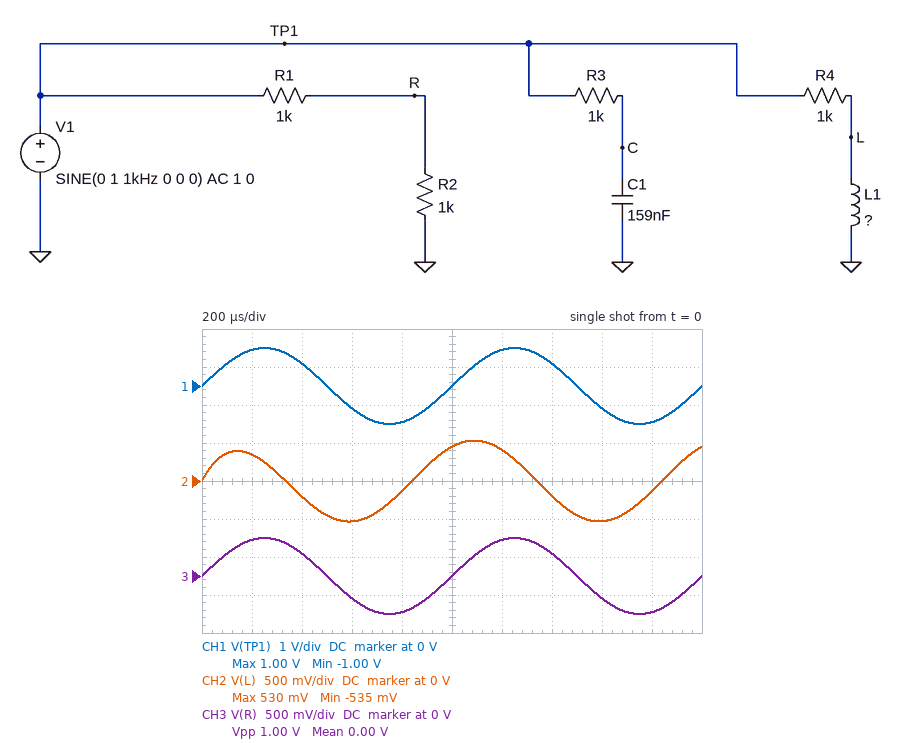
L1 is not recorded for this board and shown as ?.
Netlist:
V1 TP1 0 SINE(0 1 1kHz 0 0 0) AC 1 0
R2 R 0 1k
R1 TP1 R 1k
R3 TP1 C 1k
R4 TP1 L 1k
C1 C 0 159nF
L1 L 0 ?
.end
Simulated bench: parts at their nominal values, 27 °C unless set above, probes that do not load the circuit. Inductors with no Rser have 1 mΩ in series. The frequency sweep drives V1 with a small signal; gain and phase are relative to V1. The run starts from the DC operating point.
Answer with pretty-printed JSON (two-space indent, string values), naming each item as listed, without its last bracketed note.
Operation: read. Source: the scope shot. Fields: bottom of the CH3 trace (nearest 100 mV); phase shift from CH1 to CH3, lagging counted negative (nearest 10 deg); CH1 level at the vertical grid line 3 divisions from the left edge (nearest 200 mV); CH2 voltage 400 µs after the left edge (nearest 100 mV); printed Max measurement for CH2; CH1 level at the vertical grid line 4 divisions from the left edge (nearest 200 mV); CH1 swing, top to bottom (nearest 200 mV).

{
  "bottom of the CH3 trace": "-500 mV",
  "phase shift from CH1 to CH3, lagging counted negative": "0 deg",
  "CH1 level at the vertical grid line 3 divisions from the left edge": "-600 mV",
  "CH2 voltage 400 µs after the left edge": "-200 mV",
  "printed Max measurement for CH2": "530 mV",
  "CH1 level at the vertical grid line 4 divisions from the left edge": "-1.0 V",
  "CH1 swing, top to bottom": "2.0 V"
}
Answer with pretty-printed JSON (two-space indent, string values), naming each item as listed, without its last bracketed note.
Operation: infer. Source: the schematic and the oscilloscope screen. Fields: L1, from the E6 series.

{
  "L1, from the E6 series": "100 mH"
}
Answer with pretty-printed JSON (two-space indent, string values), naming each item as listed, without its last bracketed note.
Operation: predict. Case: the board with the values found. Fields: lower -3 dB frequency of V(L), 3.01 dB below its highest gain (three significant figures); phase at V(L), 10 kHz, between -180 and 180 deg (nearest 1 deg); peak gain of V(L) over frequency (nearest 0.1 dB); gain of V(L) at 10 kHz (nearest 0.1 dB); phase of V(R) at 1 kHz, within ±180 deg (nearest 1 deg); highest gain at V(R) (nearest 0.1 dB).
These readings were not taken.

{
  "lower -3 dB frequency of V(L), 3.01 dB below its highest gain": "1.59 kHz",
  "phase at V(L), 10 kHz, between -180 and 180 deg": "9 deg",
  "peak gain of V(L) over frequency": "0 dB",
  "gain of V(L) at 10 kHz": "-0.1 dB",
  "phase of V(R) at 1 kHz, within ±180 deg": "0 deg",
  "highest gain at V(R)": "-6.0 dB"
}
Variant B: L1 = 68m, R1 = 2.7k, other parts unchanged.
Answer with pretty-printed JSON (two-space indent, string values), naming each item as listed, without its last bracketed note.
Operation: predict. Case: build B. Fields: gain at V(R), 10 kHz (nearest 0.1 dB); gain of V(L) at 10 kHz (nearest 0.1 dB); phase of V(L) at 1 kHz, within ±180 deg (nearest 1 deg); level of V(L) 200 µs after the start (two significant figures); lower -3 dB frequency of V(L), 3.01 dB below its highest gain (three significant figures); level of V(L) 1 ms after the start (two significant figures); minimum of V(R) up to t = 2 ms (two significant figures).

{
  "gain at V(R), 10 kHz": "-11.4 dB",
  "gain of V(L) at 10 kHz": "-0.2 dB",
  "phase of V(L) at 1 kHz, within ±180 deg": "67 deg",
  "level of V(L) 200 µs after the start": "240 mV",
  "lower -3 dB frequency of V(L), 3.01 dB below its highest gain": "2.34 kHz",
  "level of V(L) 1 ms after the start": "360 mV",
  "minimum of V(R) up to t = 2 ms": "-270 mV"
}
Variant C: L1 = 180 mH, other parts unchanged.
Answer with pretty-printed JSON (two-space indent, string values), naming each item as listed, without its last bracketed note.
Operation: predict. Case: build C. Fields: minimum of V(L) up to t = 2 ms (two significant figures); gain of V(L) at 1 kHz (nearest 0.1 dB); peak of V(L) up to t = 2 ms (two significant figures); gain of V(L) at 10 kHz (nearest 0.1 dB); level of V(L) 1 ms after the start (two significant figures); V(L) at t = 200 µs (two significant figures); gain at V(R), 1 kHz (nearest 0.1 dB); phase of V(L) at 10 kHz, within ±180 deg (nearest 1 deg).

{
  "minimum of V(L) up to t = 2 ms": "-760 mV",
  "gain of V(L) at 1 kHz": "-2.5 dB",
  "peak of V(L) up to t = 2 ms": "750 mV",
  "gain of V(L) at 10 kHz": "0 dB",
  "level of V(L) 1 ms after the start": "490 mV",
  "V(L) at t = 200 µs": "520 mV",
  "gain at V(R), 1 kHz": "-6.0 dB",
  "phase of V(L) at 10 kHz, within ±180 deg": "5 deg"
}
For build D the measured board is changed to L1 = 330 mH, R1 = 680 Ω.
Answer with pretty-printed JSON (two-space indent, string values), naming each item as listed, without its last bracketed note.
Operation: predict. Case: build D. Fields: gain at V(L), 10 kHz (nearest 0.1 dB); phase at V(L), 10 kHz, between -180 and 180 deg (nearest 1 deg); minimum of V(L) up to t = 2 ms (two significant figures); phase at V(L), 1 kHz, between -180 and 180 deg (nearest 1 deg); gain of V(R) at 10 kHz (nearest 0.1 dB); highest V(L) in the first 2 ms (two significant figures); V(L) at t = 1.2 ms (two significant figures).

{
  "gain at V(L), 10 kHz": "0 dB",
  "phase at V(L), 10 kHz, between -180 and 180 deg": "3 deg",
  "minimum of V(L) up to t = 2 ms": "-950 mV",
  "phase at V(L), 1 kHz, between -180 and 180 deg": "26 deg",
  "gain of V(R) at 10 kHz": "-4.5 dB",
  "highest V(L) in the first 2 ms": "890 mV",
  "V(L) at t = 1.2 ms": "880 mV"
}
